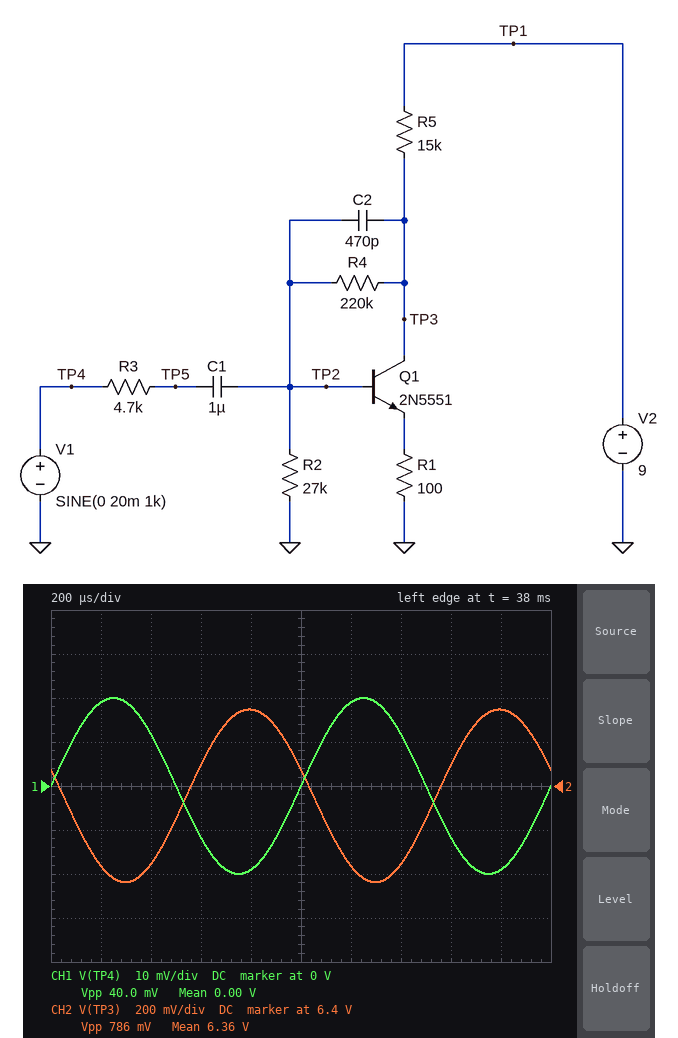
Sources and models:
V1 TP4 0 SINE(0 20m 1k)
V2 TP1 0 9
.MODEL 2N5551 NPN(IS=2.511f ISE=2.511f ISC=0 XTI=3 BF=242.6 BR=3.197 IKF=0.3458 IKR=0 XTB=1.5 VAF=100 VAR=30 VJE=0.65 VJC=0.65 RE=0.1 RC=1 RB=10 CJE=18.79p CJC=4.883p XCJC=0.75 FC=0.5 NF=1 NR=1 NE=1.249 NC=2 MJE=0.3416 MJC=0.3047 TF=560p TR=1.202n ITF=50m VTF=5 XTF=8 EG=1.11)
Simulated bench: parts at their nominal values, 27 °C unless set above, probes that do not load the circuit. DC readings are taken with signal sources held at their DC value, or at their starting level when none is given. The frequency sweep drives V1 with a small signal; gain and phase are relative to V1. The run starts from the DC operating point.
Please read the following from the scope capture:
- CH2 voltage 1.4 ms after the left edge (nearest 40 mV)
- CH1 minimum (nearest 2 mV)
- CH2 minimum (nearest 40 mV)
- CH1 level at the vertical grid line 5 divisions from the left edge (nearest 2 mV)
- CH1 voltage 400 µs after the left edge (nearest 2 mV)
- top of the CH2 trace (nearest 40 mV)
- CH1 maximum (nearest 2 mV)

6.04 V
-20 mV
5.96 V
0 V
12 mV
6.76 V
20 mV
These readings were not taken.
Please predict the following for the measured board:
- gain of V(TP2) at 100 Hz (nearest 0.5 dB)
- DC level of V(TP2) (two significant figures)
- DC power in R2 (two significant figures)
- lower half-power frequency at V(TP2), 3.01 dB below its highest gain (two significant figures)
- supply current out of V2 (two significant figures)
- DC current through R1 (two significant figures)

-8.0 dB
660 mV
16 µW
20 Hz
180 µA
150 µA
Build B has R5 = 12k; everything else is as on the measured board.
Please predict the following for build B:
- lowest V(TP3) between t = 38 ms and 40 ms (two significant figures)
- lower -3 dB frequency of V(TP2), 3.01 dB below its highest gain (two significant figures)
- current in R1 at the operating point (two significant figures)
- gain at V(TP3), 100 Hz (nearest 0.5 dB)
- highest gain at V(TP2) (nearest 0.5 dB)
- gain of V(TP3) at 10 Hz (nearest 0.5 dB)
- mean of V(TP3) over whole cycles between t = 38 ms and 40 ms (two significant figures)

6.1 V
19 Hz
180 µA
25.5 dB
-7.5 dB
19.0 dB
6.5 V
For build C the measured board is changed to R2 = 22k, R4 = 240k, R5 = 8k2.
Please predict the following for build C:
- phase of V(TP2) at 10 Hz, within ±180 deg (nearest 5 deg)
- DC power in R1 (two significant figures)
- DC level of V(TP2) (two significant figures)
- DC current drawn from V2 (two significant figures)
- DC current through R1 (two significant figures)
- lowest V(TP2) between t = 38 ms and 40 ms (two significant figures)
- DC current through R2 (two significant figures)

55 deg
1.1 µW
640 mV
130 µA
100 µA
630 mV
29 µA
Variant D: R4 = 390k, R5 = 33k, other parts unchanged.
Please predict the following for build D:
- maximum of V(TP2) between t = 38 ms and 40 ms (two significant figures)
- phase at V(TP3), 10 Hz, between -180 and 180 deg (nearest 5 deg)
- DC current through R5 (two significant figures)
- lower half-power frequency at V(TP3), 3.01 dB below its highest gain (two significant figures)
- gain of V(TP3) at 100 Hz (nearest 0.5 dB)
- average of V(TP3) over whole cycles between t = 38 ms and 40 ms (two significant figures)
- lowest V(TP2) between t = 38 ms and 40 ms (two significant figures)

550 mV
-150 deg
22 µA
6.2 Hz
7.0 dB
8.3 V
520 mV
